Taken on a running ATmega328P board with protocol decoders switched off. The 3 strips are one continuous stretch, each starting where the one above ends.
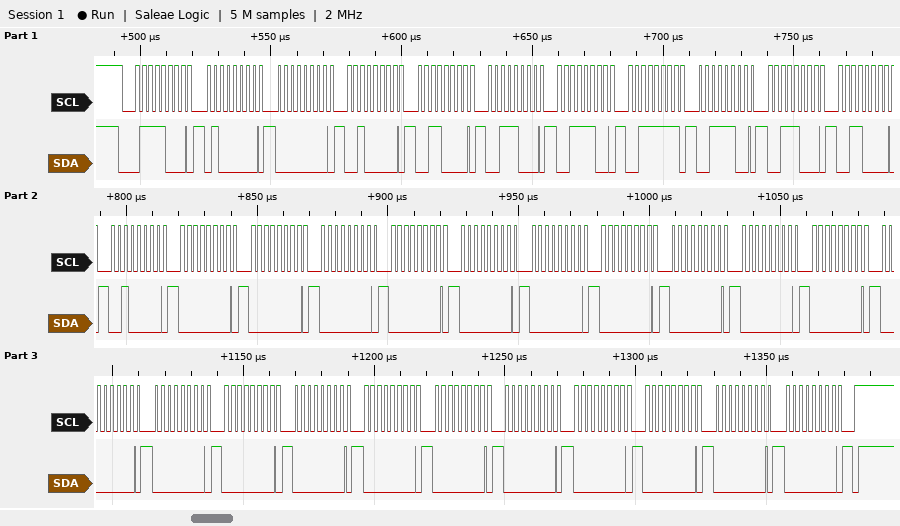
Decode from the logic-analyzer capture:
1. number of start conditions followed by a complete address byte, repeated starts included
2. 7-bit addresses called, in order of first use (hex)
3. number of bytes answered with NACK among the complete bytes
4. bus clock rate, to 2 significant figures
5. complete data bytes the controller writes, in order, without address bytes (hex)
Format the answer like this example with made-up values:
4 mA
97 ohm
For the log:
1
0x3C
0
400 kHz
40 00 20 30 38 3C 3F 3C 38 30 20 00 00 00 00 00 00 00 00 00 00 00 00 00 00 00 00 00 00 00 00 00
